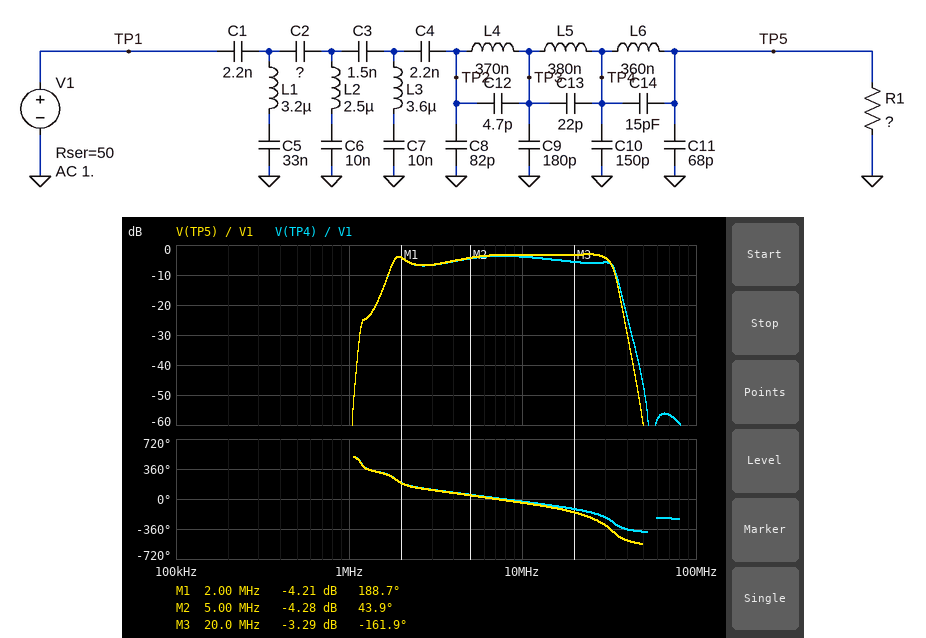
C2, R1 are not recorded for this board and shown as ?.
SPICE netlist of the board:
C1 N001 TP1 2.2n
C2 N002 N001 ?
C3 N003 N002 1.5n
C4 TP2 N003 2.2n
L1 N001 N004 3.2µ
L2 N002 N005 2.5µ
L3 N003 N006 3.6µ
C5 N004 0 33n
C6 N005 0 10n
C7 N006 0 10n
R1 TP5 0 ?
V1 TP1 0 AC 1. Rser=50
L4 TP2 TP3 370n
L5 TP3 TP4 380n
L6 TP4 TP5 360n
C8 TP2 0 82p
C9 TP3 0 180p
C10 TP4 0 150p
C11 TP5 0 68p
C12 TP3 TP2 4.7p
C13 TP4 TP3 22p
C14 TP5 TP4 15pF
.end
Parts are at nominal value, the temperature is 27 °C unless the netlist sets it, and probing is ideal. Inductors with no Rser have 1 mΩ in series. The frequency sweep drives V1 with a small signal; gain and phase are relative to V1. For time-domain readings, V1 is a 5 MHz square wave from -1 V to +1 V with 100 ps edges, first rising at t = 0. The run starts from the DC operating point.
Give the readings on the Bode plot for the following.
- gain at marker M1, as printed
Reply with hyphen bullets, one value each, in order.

- -4.21 dB
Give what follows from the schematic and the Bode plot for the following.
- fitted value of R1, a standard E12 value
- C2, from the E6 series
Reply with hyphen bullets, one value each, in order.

- 100 Ω
- 4.7 nF
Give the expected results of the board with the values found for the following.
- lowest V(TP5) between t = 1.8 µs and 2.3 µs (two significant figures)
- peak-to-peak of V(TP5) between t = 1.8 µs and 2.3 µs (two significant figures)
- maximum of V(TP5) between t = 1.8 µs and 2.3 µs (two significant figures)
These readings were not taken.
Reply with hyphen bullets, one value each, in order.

- -1.2 V
- 2.5 V
- 1.2 V
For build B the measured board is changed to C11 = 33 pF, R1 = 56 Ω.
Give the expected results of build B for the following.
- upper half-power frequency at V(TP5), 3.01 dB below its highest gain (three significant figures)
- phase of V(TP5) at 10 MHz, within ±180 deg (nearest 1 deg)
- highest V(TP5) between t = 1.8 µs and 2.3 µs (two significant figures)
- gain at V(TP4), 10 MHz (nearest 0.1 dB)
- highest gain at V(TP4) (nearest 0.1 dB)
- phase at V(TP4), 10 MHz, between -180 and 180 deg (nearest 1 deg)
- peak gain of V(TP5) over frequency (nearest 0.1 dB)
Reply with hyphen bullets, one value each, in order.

- 31.6 MHz
- -42 deg
- 980 mV
- -5.2 dB
- -2.0 dB
- -18 deg
- -5.5 dB
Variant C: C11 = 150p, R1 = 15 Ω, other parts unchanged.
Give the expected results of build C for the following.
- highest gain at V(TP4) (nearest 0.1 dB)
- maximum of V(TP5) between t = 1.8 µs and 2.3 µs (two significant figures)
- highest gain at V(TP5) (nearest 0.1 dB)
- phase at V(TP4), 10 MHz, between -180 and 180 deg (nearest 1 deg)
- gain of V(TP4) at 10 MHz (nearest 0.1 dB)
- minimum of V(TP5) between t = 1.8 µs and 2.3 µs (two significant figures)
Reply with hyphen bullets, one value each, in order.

- 3.3 dB
- 450 mV
- -11.3 dB
- 15 deg
- -8.5 dB
- -450 mV
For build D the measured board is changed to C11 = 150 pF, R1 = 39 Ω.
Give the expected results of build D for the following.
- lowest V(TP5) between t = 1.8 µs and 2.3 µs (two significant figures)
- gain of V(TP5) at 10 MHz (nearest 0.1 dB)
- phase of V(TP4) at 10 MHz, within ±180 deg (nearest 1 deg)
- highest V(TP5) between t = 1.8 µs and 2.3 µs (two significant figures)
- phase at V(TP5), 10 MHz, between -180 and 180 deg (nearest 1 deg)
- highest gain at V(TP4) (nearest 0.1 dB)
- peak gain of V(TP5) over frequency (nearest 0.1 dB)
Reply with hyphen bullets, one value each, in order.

- -820 mV
- -7.4 dB
- -15 deg
- 820 mV
- -52 deg
- 1.5 dB
- -7.1 dB
